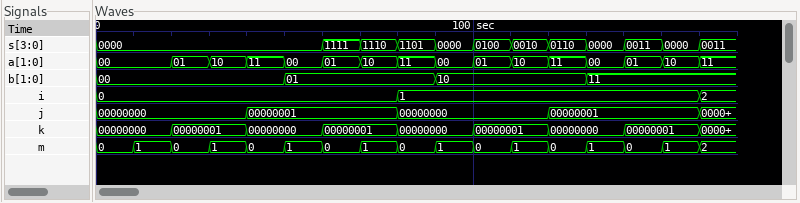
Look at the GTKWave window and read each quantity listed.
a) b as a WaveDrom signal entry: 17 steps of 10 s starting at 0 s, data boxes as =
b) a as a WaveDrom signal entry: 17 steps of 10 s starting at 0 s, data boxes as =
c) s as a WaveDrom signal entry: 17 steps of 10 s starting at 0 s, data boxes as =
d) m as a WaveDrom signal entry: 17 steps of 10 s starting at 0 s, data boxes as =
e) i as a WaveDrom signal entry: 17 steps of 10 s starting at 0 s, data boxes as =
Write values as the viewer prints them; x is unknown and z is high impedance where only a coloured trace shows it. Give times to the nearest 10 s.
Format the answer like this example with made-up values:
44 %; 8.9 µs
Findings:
{name: 'b', wave: '=....=...=...=...', data: '00 01 10 11'}; {name: 'a', wave: '=.===============', data: '00 01 10 11 00 01 10 11 00 01 10 11 00 01 10 11'}; {name: 's', wave: '=.....===========', data: '0000 1111 1110 1101 0000 0100 0010 0110 0000 0011 0000 0011'}; {name: 'm', wave: '=================', data: '0 1 0 1 0 1 0 1 0 1 0 1 0 1 0 1 2'}; {name: 'i', wave: '=.......=.......=', data: '0 1 2'}
